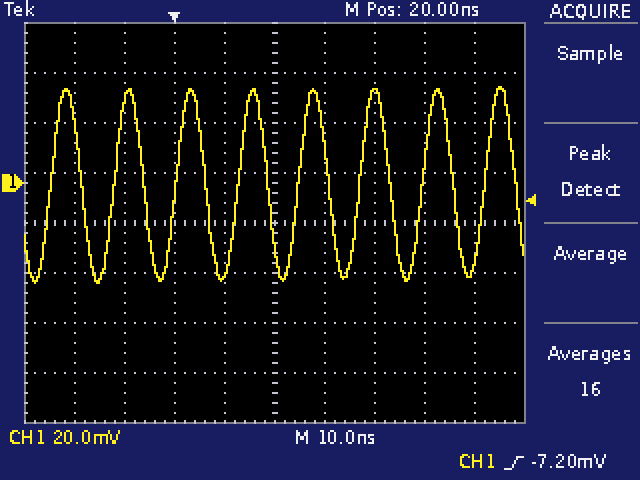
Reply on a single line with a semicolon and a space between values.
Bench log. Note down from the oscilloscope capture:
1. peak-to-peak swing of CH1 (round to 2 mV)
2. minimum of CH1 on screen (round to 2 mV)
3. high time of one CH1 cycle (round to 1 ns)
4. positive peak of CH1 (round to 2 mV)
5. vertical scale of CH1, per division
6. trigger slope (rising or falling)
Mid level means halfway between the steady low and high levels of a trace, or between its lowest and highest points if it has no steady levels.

78 mV; -40 mV; 6 ns; 38 mV; 20 mV; rising
